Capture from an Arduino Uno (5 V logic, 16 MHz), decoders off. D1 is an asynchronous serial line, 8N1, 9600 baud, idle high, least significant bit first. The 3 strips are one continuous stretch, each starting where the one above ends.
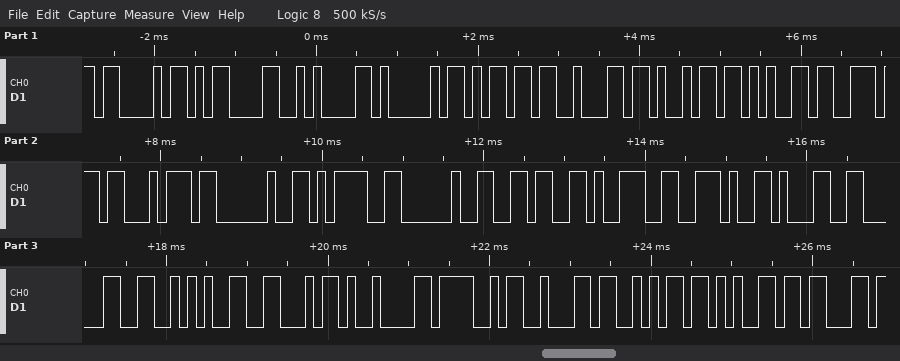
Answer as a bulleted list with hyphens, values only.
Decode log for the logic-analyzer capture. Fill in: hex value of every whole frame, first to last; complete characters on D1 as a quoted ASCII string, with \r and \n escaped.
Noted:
- 0x43 0x0D 0x0A 0x41 0x6D 0x62 0x69 0x65 0x6E 0x74 0x20 0x3D 0x20 0x36 0x39 0x2E 0x31 0x30 0x2A 0x46 0x09 0x4F 0x62 0x6A 0x65 0x63
- "C\r\nAmbient = 69.10*F\tObjec"
